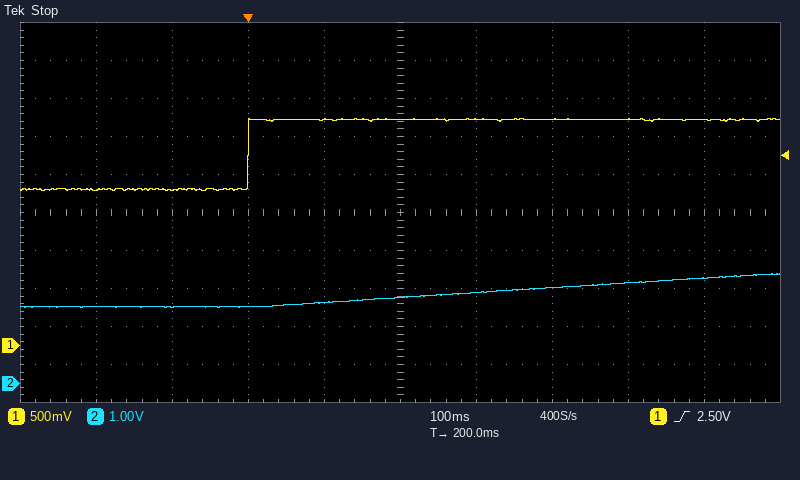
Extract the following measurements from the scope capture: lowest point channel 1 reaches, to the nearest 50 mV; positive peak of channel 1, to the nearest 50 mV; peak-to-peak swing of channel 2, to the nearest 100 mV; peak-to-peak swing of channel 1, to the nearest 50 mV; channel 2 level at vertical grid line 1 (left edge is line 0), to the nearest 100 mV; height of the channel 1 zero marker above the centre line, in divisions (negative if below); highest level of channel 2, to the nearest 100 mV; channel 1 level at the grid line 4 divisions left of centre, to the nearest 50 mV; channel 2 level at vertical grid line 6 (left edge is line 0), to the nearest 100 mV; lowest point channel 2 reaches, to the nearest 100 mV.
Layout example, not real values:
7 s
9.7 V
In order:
2.05 V
3.00 V
900 mV
950 mV
2.0 V
-3.5 div
2.9 V
2.05 V
2.4 V
2.0 V
